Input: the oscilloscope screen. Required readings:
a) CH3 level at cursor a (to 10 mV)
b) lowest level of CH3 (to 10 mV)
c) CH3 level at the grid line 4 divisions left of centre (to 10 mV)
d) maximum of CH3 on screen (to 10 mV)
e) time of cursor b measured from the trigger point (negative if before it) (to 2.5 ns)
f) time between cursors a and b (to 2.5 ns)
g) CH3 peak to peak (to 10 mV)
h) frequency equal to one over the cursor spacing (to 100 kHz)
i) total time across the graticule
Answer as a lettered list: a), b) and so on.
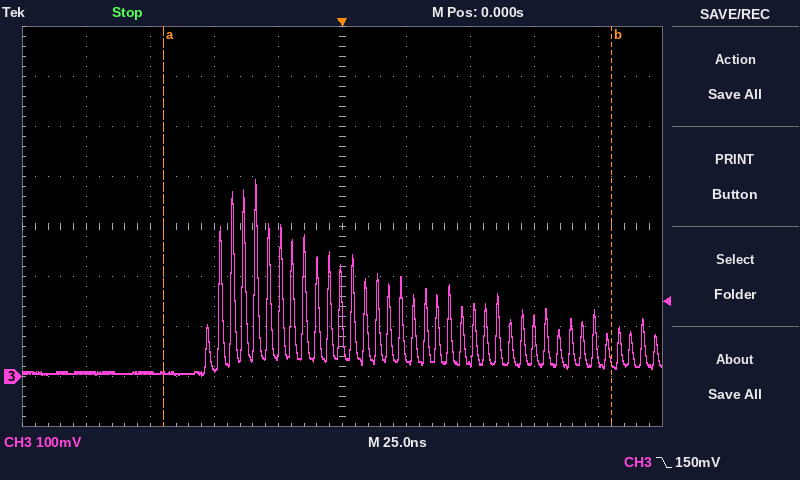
a) 10 mV
b) 0 mV
c) 10 mV
d) 390 mV
e) +105.0 ns
f) 175.0 ns
g) 390 mV
h) 5.7 MHz
i) 250 ns
